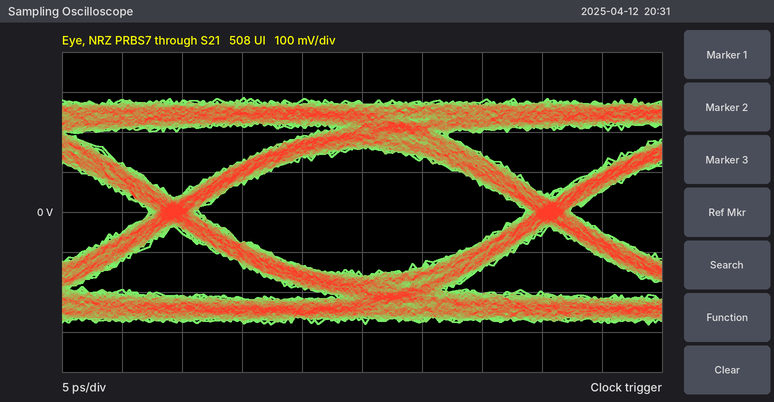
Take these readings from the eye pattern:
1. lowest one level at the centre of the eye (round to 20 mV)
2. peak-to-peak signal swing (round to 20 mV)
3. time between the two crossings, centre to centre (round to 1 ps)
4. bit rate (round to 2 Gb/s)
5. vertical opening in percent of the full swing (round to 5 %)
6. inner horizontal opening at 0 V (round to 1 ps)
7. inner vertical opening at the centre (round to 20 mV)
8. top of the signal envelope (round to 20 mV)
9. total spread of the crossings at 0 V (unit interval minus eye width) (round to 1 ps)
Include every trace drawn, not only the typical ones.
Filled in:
160 mV
560 mV
31 ps
32 Gb/s
55 %
27 ps
320 mV
280 mV
4 ps
